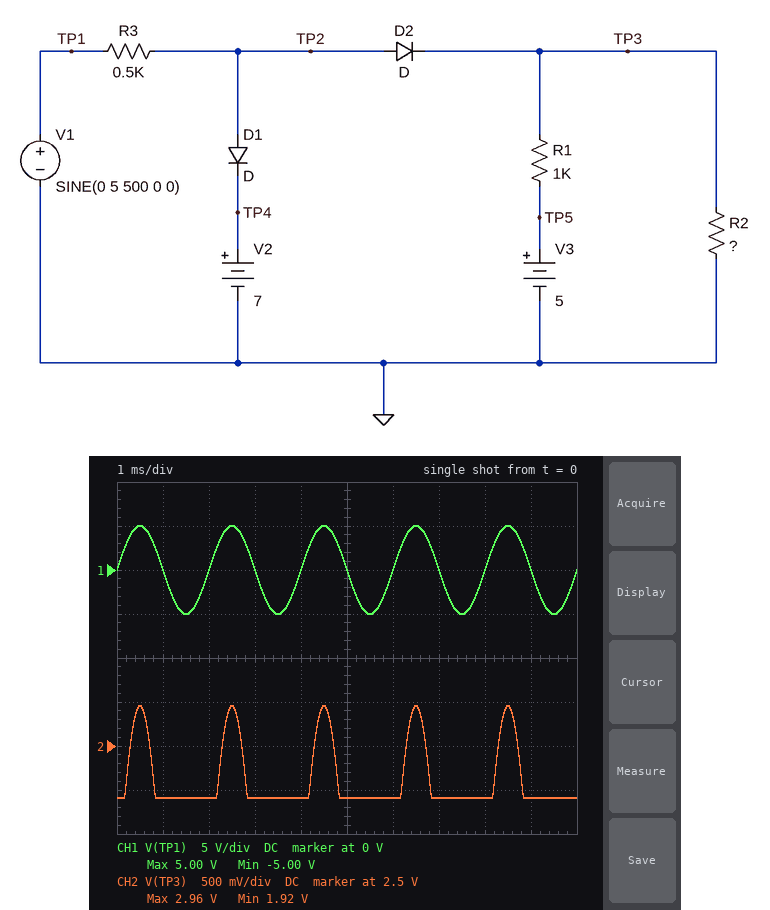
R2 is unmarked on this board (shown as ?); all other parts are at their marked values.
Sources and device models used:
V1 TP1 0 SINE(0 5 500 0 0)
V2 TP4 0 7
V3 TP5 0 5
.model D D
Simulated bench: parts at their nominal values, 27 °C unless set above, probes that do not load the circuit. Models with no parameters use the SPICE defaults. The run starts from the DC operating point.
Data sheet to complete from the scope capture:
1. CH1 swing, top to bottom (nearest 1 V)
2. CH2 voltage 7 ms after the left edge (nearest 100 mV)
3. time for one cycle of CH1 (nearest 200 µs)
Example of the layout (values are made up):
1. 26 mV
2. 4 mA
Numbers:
1. 10 V
2. 1.9 V
3. 2.0 ms
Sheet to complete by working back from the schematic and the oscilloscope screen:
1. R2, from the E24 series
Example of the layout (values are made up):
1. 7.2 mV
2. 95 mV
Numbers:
1. 620 Ω
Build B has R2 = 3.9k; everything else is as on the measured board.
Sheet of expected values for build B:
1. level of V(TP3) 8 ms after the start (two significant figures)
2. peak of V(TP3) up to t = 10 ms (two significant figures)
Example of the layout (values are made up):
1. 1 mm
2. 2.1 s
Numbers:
1. 4.0 V
2. 4.2 V
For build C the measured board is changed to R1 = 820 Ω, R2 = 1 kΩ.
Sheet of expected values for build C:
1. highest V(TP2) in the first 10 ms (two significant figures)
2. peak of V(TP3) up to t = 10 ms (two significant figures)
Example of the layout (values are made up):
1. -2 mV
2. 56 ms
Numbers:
1. 4.2 V
2. 3.5 V
